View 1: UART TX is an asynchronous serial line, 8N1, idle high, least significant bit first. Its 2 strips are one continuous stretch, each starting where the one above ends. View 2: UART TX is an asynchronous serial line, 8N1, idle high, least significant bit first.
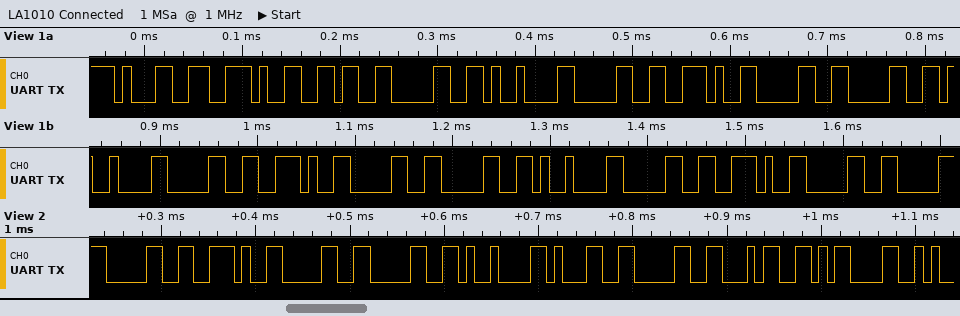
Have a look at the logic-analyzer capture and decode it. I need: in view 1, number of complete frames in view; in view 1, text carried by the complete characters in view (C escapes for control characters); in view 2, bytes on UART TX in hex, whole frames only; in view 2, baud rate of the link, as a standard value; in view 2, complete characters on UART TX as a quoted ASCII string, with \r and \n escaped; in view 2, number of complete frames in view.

18
"1.60\t0.00\t0.00\t0.0"
0x30 0x2E 0x30 0x30 0x09 0x31 0x30 0x34 0x0D
115200 baud
"0.00\t104\r"
9
